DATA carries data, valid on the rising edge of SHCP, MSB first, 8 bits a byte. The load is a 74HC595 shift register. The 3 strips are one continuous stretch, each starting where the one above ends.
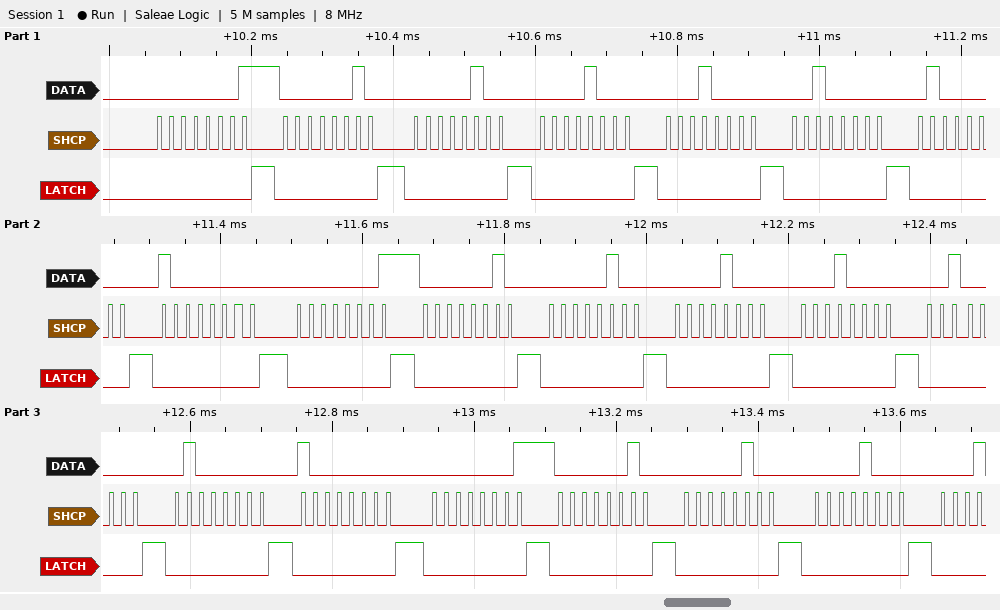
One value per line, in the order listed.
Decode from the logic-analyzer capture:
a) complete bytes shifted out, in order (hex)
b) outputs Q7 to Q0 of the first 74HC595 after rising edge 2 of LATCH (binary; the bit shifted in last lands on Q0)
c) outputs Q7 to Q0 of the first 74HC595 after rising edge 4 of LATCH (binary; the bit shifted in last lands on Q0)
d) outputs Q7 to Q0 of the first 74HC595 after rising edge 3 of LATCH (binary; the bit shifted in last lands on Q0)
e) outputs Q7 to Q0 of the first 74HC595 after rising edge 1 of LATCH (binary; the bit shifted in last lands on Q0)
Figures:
01 02 04 08 10 20 40 80 01 02 04 08 10 20 40 80 01 02 04 08
00000010
00001000
00000100
00000001
